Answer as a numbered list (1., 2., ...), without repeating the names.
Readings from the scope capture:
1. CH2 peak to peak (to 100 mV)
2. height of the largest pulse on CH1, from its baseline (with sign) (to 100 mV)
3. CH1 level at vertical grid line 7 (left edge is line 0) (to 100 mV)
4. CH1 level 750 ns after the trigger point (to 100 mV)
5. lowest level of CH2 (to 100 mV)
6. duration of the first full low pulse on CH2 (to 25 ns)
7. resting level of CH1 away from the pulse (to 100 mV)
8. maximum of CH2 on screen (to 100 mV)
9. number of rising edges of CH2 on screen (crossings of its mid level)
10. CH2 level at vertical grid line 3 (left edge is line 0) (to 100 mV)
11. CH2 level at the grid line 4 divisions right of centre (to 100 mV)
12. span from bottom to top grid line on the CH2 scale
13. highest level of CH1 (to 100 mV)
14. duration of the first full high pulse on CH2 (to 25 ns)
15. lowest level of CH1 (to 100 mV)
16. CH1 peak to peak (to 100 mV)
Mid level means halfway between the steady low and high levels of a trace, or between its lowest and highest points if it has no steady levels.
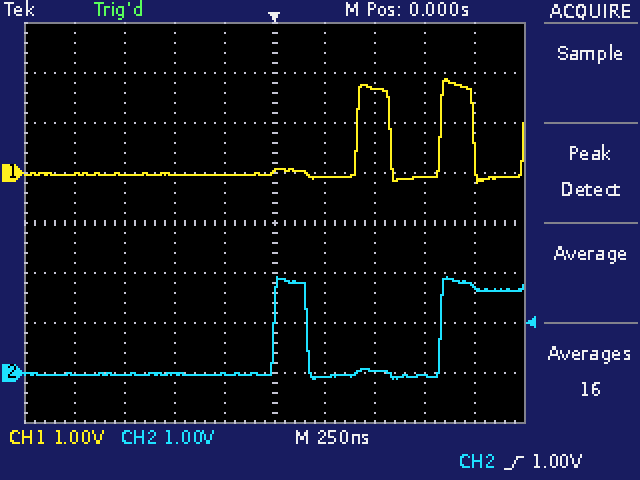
1. 2.0 V
2. +1.9 V
3. 1.7 V
4. -100 mV
5. -100 mV
6. 675 ns
7. 0.0 V
8. 1.9 V
9. 2
10. 0.0 V
11. 1.7 V
12. 8 V
13. 1.9 V
14. 175 ns
15. -200 mV
16. 2.1 V
